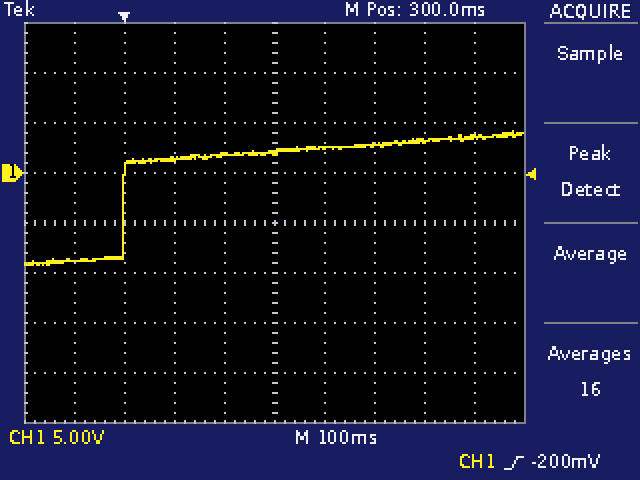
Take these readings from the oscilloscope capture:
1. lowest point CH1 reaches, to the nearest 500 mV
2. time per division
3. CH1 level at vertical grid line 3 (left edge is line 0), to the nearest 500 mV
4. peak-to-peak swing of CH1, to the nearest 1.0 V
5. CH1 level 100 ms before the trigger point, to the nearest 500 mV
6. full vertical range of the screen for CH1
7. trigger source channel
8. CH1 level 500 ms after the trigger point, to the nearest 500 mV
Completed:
-9.0 V
100 ms
1.5 V
13.0 V
-9.0 V
40 V
CH1
3.0 V
